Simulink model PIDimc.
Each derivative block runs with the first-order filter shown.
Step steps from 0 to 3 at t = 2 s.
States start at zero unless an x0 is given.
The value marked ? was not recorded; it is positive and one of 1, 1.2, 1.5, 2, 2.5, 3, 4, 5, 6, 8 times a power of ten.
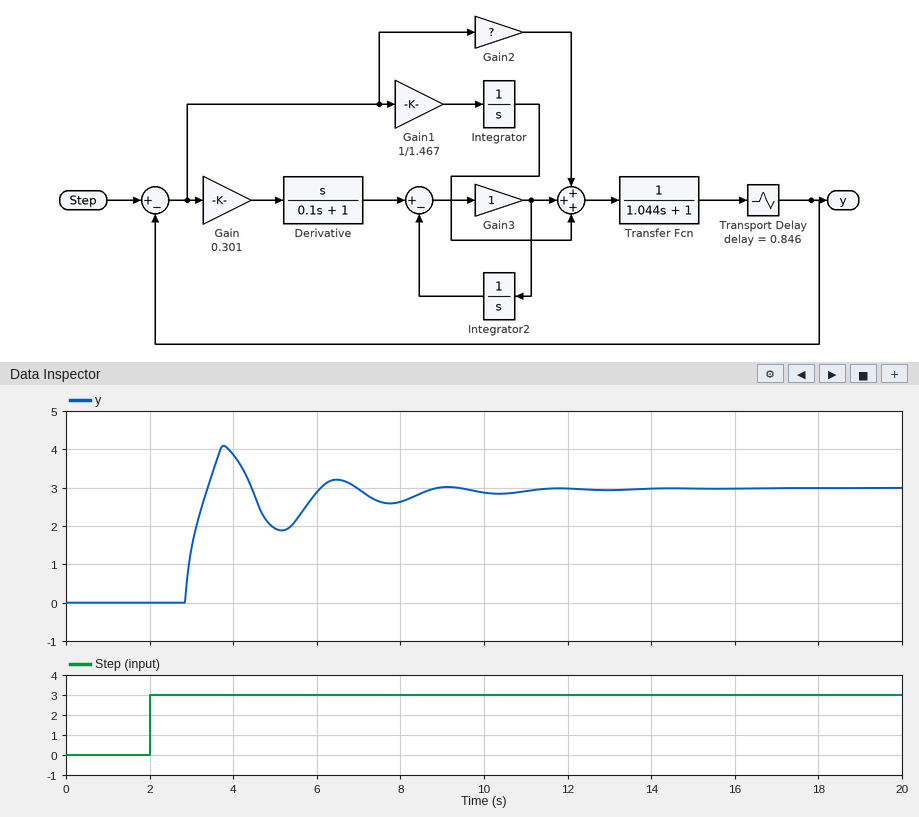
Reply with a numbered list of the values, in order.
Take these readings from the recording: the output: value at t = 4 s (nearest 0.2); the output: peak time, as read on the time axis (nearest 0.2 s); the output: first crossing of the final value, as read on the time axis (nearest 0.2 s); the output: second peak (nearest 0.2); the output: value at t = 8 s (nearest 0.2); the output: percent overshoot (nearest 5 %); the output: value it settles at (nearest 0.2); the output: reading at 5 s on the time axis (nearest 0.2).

1. 3.8
2. 3.8 s
3. 3.4 s
4. 3.2
5. 2.6
6. 35 %
7. 3.0
8. 2.0
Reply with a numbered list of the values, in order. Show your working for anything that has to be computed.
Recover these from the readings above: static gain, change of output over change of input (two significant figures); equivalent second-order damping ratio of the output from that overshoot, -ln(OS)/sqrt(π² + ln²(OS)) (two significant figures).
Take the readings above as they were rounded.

1. (3 - 0) / (3 - 0) = 1.0
2. ln(0.35) = -1.050; 1.050 / sqrt(9.870 + 1.102) = 0.32
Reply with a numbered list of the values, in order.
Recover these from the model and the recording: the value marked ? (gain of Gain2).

1. 2
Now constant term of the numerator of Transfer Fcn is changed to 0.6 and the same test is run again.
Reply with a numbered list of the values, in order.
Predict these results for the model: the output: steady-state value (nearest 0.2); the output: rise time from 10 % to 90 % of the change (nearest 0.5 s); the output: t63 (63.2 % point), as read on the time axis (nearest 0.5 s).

1. 3.0
2. 5.5 s
3. 3.5 s
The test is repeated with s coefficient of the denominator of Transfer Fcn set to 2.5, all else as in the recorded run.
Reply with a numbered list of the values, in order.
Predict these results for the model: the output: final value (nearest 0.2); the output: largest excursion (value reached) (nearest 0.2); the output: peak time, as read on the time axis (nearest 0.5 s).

1. 3.0
2. 3.2
3. 5.5 s
